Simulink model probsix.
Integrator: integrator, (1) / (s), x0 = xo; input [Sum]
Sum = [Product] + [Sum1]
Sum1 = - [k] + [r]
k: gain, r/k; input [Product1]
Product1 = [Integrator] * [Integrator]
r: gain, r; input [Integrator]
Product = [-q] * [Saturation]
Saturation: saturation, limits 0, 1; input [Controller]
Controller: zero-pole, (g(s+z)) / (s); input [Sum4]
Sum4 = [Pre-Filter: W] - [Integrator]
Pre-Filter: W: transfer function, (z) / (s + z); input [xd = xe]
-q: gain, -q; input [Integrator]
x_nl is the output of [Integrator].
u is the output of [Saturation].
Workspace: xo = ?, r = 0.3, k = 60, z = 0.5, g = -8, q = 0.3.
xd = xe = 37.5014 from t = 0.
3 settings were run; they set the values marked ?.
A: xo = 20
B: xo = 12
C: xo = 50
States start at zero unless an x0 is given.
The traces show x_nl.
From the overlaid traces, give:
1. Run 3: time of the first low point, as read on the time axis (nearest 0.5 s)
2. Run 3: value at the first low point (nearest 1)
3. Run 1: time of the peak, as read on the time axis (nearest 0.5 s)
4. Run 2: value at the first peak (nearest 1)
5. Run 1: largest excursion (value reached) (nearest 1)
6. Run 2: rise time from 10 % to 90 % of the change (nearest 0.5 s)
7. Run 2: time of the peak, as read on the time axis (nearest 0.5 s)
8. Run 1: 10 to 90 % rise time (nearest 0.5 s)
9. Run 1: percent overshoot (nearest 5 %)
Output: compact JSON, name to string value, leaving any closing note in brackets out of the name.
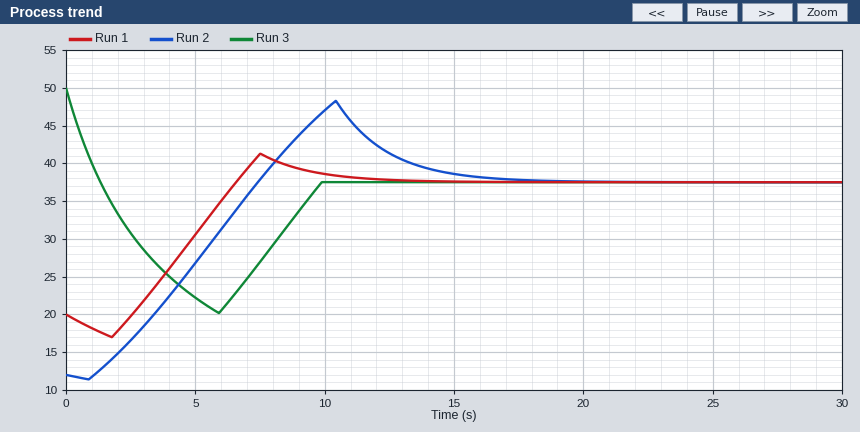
{"Run 3: time of the first low point, as read on the time axis": "6.0 s", "Run 3: value at the first low point": "20", "Run 1: time of the peak, as read on the time axis": "7.5 s", "Run 2: value at the first peak": "48", "Run 1: largest excursion (value reached)": "41", "Run 2: rise time from 10 % to 90 % of the change": "5.0 s", "Run 2: time of the peak, as read on the time axis": "10.5 s", "Run 1: 10 to 90 % rise time": "3.0 s", "Run 1: percent overshoot": "20 %"}
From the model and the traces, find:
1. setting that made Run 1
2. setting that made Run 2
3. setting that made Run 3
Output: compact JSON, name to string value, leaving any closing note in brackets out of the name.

{"setting that made Run 1": "A", "setting that made Run 2": "B", "setting that made Run 3": "C"}
